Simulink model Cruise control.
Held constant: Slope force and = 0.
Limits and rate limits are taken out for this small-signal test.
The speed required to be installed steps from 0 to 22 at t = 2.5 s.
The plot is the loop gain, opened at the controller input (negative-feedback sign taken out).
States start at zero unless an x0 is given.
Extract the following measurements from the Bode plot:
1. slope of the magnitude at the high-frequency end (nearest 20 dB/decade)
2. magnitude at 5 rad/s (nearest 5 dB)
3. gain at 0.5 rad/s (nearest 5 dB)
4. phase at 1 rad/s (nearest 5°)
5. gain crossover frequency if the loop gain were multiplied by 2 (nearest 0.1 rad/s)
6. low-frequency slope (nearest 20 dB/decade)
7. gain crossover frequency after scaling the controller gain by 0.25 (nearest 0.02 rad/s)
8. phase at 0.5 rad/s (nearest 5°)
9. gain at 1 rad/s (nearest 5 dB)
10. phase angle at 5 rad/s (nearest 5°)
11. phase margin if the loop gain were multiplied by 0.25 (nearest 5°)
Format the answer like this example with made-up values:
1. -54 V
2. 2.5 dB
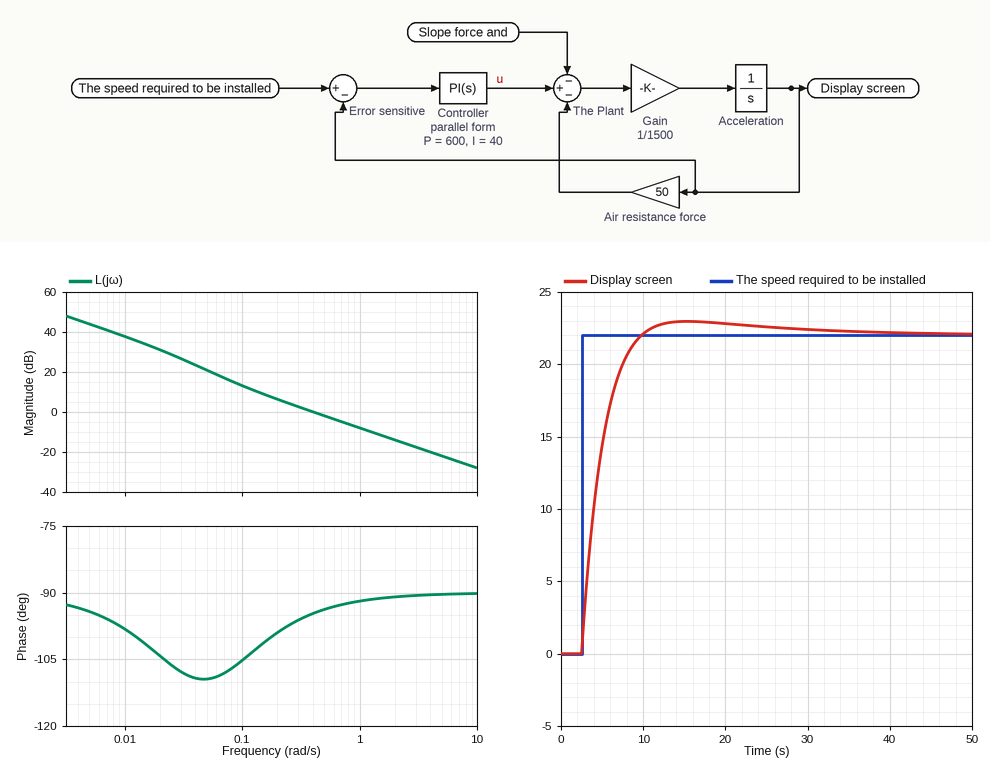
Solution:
1. -20 dB/decade
2. -20 dB
3. 0 dB
4. -90°
5. 0.8 rad/s
6. -20 dB/decade
7. 0.12 rad/s
8. -95°
9. -10 dB
10. -90°
11. 75°
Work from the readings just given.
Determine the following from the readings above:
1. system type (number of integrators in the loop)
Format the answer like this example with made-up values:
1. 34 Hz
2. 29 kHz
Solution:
1. 1
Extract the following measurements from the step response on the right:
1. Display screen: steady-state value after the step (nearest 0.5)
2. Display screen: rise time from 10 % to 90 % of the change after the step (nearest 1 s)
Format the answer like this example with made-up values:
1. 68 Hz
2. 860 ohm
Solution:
1. 22.0
2. 5 s
